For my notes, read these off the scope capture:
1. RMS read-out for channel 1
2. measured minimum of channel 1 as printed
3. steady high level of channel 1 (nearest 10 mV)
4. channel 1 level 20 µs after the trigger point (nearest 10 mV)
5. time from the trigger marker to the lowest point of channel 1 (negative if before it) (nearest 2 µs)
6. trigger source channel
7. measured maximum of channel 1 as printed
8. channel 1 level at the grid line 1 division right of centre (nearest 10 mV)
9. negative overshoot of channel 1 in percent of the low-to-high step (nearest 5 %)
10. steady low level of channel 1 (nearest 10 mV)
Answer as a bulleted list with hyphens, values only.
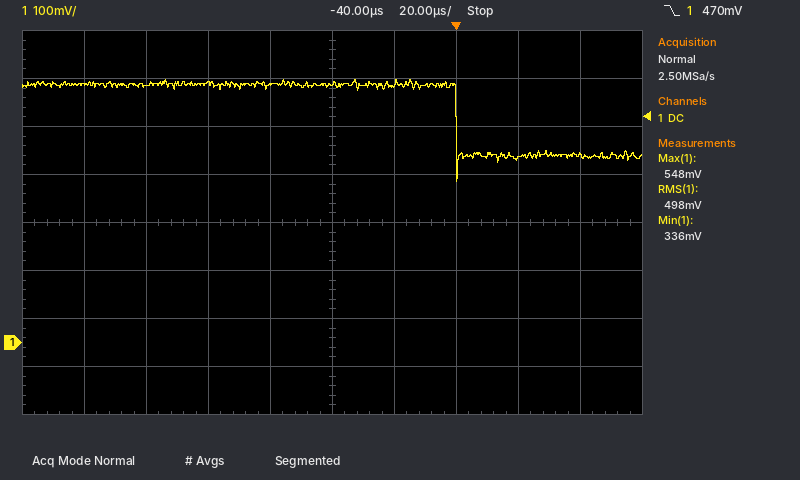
- 498 mV
- 336 mV
- 540 mV
- 380 mV
- 0 µs
- channel 1
- 548 mV
- 540 mV
- 35 %
- 390 mV
